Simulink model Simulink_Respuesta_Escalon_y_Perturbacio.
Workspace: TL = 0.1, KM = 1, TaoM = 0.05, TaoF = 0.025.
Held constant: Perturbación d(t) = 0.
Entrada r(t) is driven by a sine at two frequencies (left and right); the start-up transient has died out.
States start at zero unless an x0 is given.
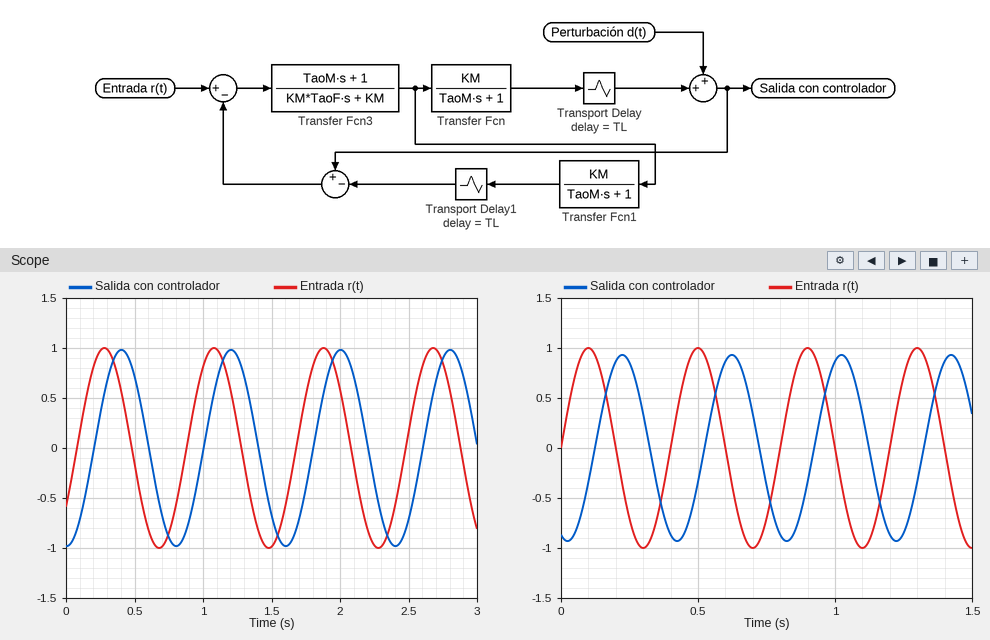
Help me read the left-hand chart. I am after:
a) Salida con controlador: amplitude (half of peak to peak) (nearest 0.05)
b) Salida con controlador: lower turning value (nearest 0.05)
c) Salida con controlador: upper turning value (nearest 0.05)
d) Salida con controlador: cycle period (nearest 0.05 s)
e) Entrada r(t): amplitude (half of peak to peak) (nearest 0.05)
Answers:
1.00
-1.00
1.00
0.80 s
1.00
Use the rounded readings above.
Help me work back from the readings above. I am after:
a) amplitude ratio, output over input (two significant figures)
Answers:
1.0
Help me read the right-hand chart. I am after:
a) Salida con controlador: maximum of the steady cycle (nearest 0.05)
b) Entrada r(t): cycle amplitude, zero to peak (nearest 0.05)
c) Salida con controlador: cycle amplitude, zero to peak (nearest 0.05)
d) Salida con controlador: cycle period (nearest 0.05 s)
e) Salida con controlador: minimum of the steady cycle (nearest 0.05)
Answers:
0.95
1.00
0.95
0.40 s
-0.95
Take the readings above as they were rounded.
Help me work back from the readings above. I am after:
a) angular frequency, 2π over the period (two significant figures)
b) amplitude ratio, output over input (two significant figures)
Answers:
16 rad/s
0.95
